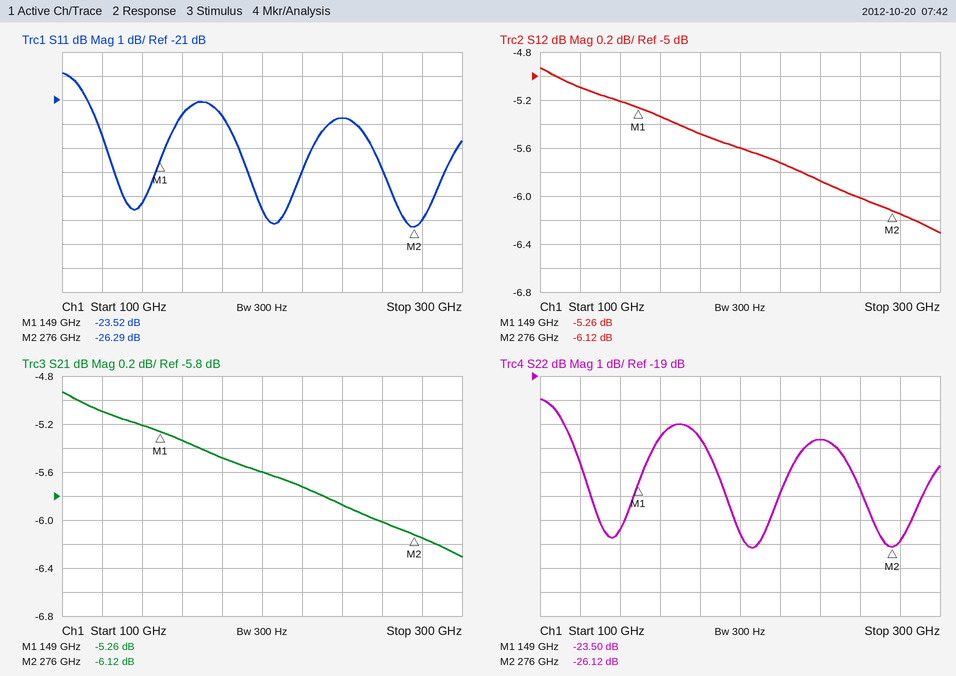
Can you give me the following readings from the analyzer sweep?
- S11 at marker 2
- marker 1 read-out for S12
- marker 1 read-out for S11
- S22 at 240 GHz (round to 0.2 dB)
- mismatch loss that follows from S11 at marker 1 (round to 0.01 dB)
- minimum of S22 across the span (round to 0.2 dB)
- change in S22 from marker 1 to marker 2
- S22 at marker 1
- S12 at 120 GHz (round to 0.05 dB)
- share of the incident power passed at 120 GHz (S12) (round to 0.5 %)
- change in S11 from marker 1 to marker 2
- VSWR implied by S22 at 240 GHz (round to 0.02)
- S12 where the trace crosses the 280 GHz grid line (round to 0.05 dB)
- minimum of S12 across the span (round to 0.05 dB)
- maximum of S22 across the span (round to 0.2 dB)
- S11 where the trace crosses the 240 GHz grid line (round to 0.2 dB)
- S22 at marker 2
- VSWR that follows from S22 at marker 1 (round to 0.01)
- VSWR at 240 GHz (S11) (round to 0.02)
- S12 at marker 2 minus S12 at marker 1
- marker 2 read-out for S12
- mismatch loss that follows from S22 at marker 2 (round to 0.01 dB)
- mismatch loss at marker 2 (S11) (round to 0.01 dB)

-26.29 dB
-5.26 dB
-23.52 dB
-21.6 dB
0.02 dB
-26.2 dB
-2.62 dB
-23.50 dB
-5.10 dB
31.0 %
-2.77 dB
1.18
-6.15 dB
-6.30 dB
-20.0 dB
-21.8 dB
-26.12 dB
1.14
1.18
-0.86 dB
-6.12 dB
0.01 dB
0.01 dB
